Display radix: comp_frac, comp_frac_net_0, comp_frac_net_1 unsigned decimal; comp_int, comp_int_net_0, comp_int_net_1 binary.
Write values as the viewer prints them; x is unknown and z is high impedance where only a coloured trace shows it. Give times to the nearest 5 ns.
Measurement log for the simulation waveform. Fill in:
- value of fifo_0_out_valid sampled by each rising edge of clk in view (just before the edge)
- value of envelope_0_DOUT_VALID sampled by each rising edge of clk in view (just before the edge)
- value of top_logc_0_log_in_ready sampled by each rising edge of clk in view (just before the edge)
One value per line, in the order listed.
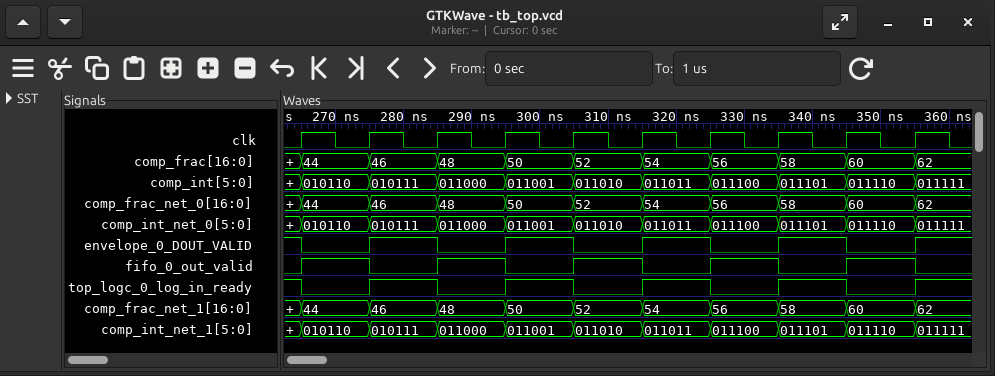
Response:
0 1 0 1 0 1 0 1 0 1
1 0 1 0 1 0 1 0 1 0
1 0 1 0 1 0 1 0 1 0
